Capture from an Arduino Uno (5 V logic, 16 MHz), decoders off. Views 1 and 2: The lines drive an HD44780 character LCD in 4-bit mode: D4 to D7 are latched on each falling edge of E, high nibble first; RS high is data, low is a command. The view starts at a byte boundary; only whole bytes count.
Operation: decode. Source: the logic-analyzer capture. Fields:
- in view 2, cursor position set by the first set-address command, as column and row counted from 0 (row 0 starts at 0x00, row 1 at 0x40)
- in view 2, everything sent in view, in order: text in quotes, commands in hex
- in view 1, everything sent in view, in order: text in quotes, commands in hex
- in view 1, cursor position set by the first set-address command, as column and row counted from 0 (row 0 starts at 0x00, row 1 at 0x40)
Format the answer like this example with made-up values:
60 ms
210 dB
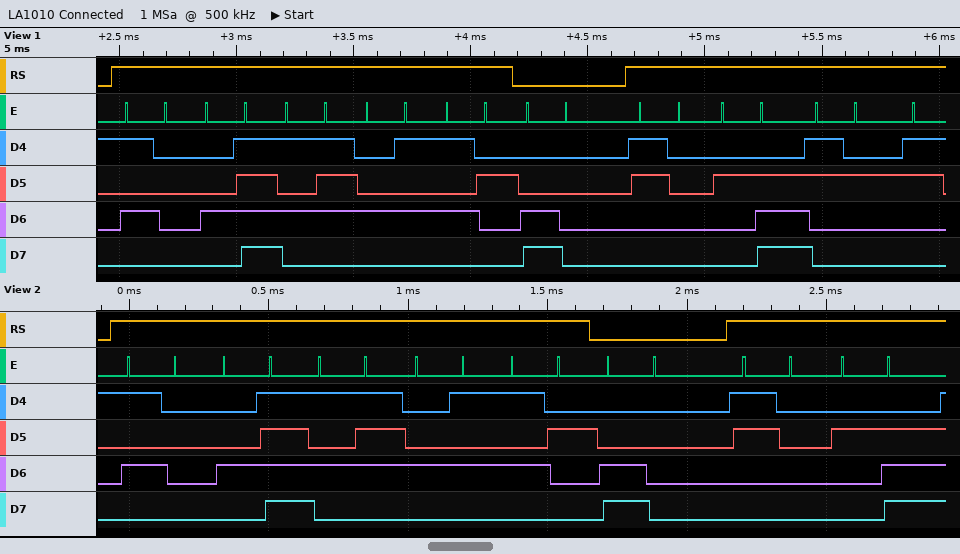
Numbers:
column 0, row 1
"POWER" 0xC0 "0."
"POWER" 0xC0 "0.2"
column 0, row 1
